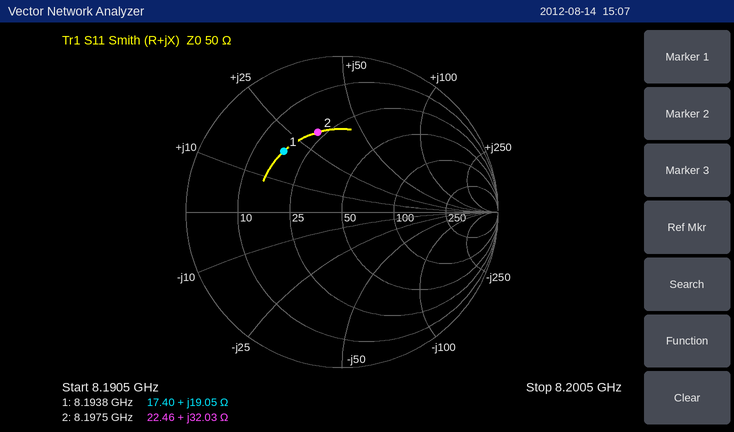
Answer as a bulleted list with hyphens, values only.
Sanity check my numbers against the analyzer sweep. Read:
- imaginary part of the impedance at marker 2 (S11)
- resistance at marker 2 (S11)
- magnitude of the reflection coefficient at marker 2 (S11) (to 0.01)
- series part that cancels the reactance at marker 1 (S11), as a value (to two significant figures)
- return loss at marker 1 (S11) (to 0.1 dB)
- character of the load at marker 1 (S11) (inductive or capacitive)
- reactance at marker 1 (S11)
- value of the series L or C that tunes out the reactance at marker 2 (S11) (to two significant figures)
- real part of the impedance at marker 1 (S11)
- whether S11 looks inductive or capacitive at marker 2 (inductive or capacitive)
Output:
- +32.03 Ω
- 22.46 Ω
- 0.53
- 1.0 pF
- 5.4 dB
- inductive
- +19.05 Ω
- 610 fF
- 17.40 Ω
- inductive
